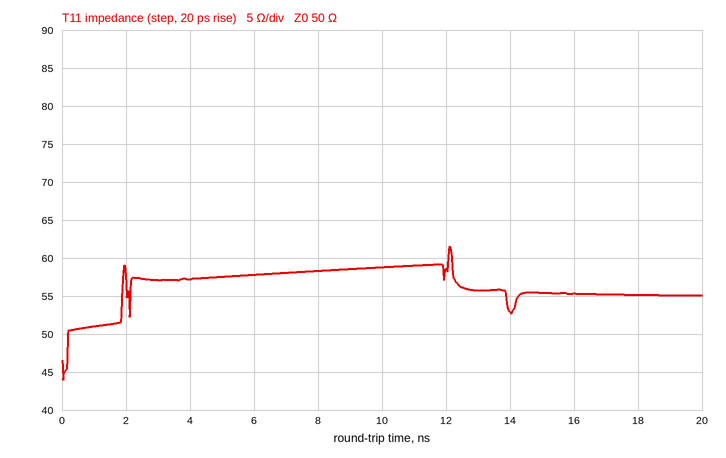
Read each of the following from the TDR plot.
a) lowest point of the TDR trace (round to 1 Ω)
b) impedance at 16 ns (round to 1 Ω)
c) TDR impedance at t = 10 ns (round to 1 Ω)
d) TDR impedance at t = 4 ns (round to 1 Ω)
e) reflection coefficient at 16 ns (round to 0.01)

44 Ω
55 Ω
59 Ω
57 Ω
+0.05
